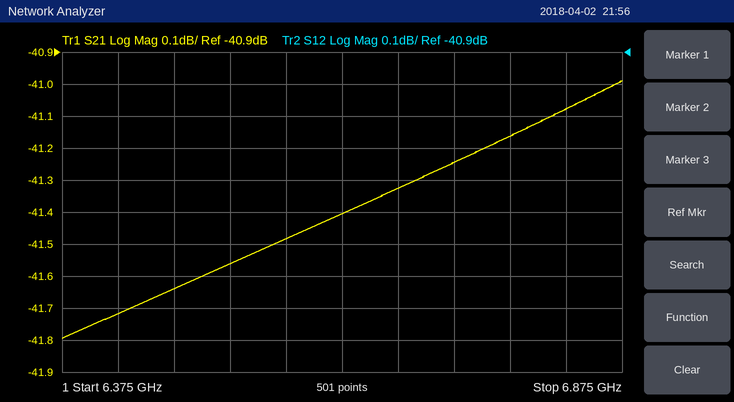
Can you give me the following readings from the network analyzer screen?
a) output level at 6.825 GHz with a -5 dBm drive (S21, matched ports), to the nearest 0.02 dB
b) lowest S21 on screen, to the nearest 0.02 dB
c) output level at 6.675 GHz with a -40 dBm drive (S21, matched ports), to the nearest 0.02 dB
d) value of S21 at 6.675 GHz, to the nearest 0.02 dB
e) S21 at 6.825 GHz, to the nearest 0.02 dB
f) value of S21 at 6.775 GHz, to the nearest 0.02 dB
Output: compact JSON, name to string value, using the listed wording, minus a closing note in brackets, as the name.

{"output level at 6.825 GHz with a -5 dBm drive (S21, matched ports), to the nearest 0.02 dB": "-46.08 dBm", "lowest S21 on screen, to the nearest 0.02 dB": "-41.80 dB", "output level at 6.675 GHz with a -40 dBm drive (S21, matched ports), to the nearest 0.02 dB": "-81.32 dBm", "value of S21 at 6.675 GHz, to the nearest 0.02 dB": "-41.32 dB", "S21 at 6.825 GHz, to the nearest 0.02 dB": "-41.08 dB", "value of S21 at 6.775 GHz, to the nearest 0.02 dB": "-41.16 dB"}
